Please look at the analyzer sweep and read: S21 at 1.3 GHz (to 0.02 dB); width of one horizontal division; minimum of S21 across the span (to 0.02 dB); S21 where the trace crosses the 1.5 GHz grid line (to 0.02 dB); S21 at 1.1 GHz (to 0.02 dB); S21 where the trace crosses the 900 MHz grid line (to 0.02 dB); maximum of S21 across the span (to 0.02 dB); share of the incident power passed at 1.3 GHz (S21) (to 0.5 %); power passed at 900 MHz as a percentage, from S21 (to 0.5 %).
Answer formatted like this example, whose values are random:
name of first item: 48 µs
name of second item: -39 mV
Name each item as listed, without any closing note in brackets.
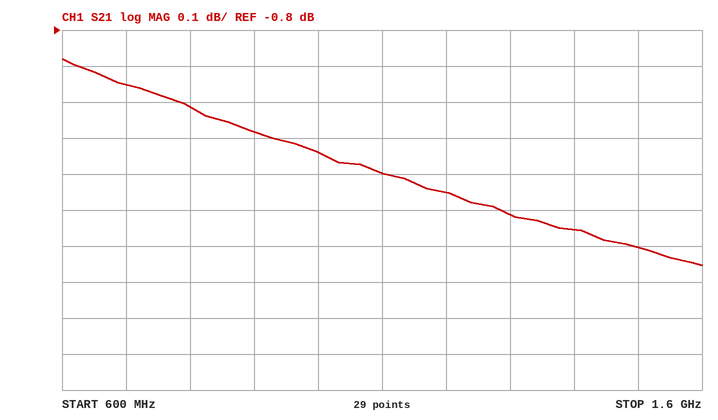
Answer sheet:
S21 at 1.3 GHz: -1.32 dB
width of one horizontal division: 100 MHz
minimum of S21 across the span: -1.46 dB
S21 where the trace crosses the 1.5 GHz grid line: -1.40 dB
S21 at 1.1 GHz: -1.20 dB
S21 where the trace crosses the 900 MHz grid line: -1.08 dB
maximum of S21 across the span: -0.88 dB
share of the incident power passed at 1.3 GHz (S21): 74.0 %
power passed at 900 MHz as a percentage, from S21: 78.0 %
